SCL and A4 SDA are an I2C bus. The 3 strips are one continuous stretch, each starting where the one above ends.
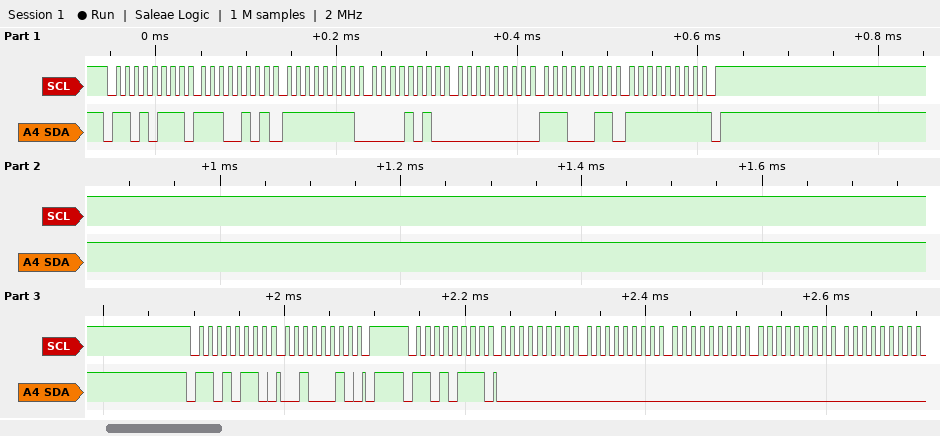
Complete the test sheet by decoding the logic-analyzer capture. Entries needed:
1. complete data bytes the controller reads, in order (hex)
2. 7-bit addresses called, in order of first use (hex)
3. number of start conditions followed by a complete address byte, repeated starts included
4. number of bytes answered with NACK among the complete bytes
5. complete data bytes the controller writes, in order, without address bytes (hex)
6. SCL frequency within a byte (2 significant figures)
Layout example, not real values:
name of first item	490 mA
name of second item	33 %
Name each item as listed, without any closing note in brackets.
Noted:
complete data bytes the controller reads, in order	E5 FF 0A 00 E3 FF 00 00 00 00 00
7-bit addresses called, in order of first use	0x6B
number of start conditions followed by a complete address byte, repeated starts included	3
number of bytes answered with NACK among the complete bytes	1
complete data bytes the controller writes, in order, without address bytes	22
SCL frequency within a byte	100 kHz
